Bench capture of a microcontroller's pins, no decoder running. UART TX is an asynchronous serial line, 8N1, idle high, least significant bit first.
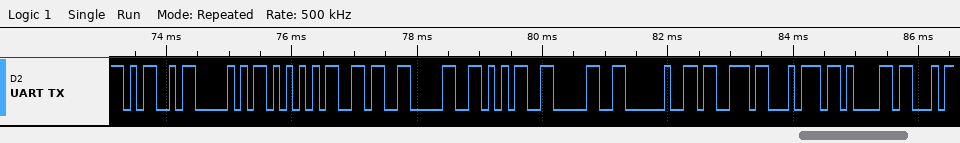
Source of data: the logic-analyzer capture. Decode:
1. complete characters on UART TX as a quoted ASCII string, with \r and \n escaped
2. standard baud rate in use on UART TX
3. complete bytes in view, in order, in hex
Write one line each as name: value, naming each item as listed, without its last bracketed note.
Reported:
complete characters on UART TX as a quoted ASCII string, with \r and \n escaped: "MPU6050 sta"
standard baud rate in use on UART TX: 9600 baud
complete bytes in view, in order, in hex: 4D 50 55 36 30 35 30 20 73 74 61
